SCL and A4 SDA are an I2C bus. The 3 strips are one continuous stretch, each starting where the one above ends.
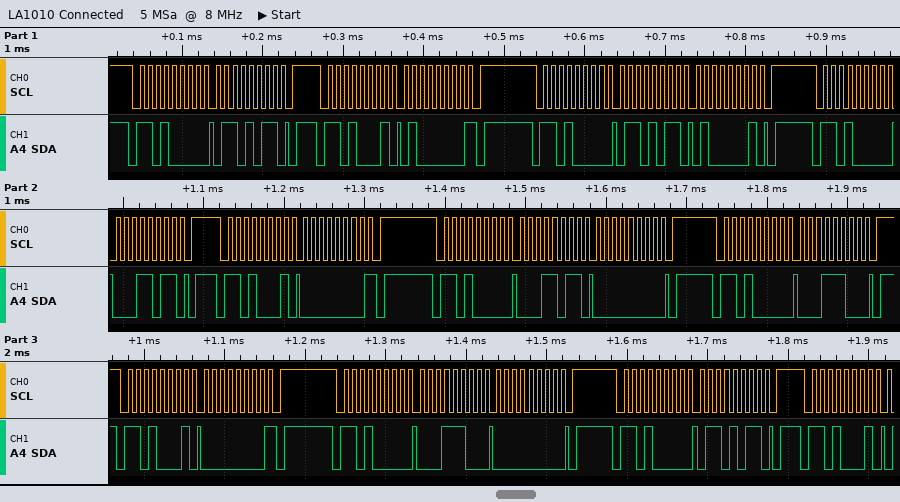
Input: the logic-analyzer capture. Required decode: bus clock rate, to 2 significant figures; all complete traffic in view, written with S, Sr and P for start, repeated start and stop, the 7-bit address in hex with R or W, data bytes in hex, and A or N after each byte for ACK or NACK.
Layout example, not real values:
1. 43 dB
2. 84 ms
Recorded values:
1. 100 kHz
2. S 68W A 6B A P S 68R A 40 N P S 68W A 6B A 41 A P S 68W A 1B A P S 68R A 00 N P S 68W A 1B A 00 A P S 68W A 1C A P S 68R A 00 N P S 68W A 1C A 00 A P S 68W A 6B A P S 68R A
